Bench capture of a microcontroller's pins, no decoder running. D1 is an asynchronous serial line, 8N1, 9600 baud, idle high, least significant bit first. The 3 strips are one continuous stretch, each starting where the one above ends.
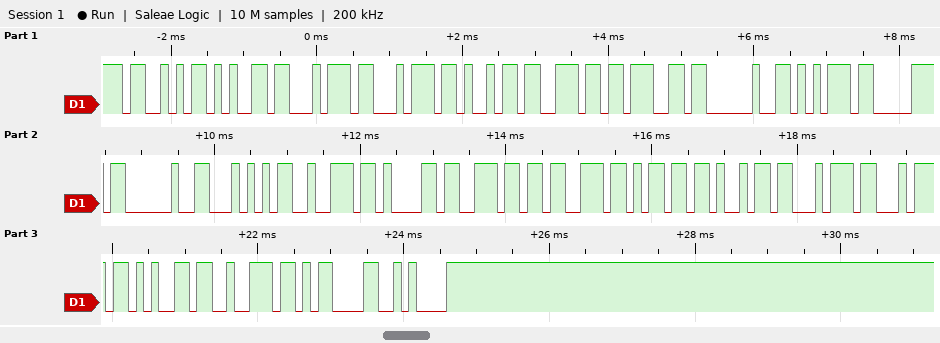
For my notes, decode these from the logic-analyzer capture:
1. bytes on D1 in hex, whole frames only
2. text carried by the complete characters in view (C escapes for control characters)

53 65 74 74 69 6E 67 20 75 70 20 54 72 61 6E 73 6D 69 74 74 65 72 0D 0A
"Setting up Transmitter\r\n"
